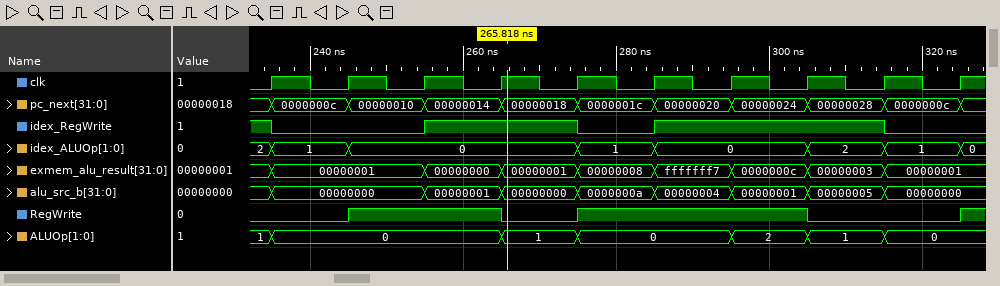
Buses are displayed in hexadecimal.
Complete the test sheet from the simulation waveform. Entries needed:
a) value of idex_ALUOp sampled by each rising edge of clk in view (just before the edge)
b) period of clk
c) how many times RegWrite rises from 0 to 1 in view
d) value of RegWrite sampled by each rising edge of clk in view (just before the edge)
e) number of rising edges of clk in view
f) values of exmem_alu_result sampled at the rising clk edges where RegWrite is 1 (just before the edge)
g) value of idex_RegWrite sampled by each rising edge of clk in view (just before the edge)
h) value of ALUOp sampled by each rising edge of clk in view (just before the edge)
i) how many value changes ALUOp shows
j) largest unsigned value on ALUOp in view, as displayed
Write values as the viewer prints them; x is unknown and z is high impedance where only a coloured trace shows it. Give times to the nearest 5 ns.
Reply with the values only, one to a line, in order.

2, 1, 0, 0, 0, 1, 0, 0, 2, 1
10 ns
3
0 0 1 1 0 1 1 1 0 0
10
00000001, 00000000, 00000008, fffffff7, 0000000c
1 0 0 1 1 0 1 1 1 0
1, 0, 0, 0, 1, 0, 0, 2, 1, 0
6
2
